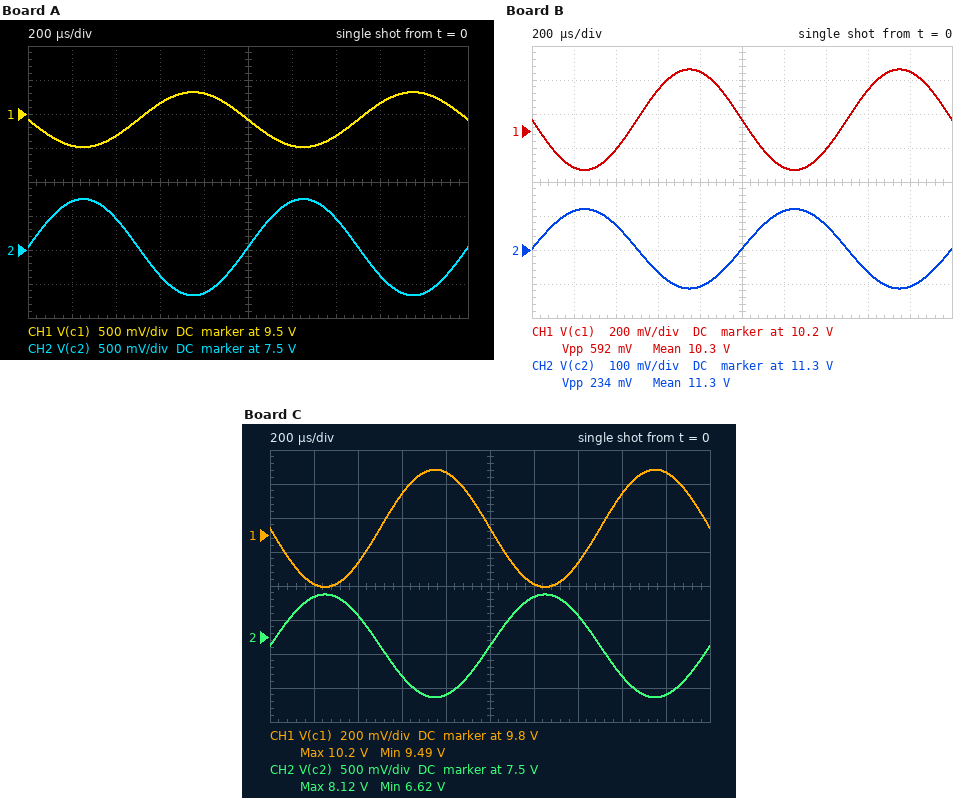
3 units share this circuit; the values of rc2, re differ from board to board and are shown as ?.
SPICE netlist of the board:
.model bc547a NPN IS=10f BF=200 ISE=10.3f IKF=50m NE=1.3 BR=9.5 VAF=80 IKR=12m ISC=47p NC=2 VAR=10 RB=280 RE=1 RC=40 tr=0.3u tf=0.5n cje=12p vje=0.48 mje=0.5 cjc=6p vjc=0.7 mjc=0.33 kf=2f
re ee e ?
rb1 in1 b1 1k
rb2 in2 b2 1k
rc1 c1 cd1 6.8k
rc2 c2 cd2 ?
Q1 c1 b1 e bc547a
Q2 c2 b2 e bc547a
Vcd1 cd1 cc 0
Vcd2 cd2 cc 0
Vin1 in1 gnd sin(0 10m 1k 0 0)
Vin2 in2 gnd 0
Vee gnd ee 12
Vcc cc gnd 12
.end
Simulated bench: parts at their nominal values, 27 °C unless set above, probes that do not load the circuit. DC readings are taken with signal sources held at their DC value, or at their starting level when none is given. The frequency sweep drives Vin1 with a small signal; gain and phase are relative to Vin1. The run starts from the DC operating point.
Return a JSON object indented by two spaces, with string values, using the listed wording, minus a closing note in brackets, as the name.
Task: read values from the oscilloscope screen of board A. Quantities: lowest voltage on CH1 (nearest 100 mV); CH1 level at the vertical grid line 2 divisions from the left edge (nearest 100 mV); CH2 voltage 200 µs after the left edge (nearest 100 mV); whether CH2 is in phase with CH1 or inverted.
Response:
{
  "lowest voltage on CH1": "9.0 V",
  "CH1 level at the vertical grid line 2 divisions from the left edge": "9.2 V",
  "CH2 voltage 200 µs after the left edge": "8.2 V",
  "whether CH2 is in phase with CH1 or inverted": "inverted"
}
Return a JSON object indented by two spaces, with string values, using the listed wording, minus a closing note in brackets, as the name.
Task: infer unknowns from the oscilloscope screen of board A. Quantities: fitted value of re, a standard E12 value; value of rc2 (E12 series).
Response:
{
  "fitted value of re, a standard E12 value": "15 kΩ",
  "value of rc2": "12 kΩ"
}
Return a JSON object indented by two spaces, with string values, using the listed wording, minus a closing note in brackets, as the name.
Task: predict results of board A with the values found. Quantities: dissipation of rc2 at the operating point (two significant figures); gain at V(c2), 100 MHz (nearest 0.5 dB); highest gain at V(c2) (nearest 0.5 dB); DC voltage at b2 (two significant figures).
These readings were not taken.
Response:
{
  "dissipation of rc2 at the operating point": "1.7 mW",
  "gain at V(c2), 100 MHz": "-10.0 dB",
  "highest gain at V(c2)": "37.0 dB",
  "DC voltage at b2": "-3.2 mV"
}
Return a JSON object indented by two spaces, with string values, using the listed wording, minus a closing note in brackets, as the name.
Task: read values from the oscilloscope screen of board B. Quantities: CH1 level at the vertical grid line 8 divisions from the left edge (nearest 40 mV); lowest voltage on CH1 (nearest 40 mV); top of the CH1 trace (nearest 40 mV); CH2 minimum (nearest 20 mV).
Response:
{
  "CH1 level at the vertical grid line 8 divisions from the left edge": "10.44 V",
  "lowest voltage on CH1": "9.96 V",
  "top of the CH1 trace": "10.56 V",
  "CH2 minimum": "11.18 V"
}
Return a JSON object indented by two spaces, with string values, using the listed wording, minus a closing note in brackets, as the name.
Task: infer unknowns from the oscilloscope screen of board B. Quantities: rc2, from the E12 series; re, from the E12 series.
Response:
{
  "rc2, from the E12 series": "2.7 kΩ",
  "re, from the E12 series": "22 kΩ"
}
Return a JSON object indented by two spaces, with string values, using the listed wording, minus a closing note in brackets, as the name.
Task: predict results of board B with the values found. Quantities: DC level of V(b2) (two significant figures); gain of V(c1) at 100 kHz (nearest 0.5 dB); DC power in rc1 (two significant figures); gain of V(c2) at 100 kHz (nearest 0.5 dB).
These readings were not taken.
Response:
{
  "DC level of V(b2)": "-2.2 mV",
  "gain of V(c1) at 100 kHz": "29.5 dB",
  "DC power in rc1": "440 µW",
  "gain of V(c2) at 100 kHz": "21.5 dB"
}
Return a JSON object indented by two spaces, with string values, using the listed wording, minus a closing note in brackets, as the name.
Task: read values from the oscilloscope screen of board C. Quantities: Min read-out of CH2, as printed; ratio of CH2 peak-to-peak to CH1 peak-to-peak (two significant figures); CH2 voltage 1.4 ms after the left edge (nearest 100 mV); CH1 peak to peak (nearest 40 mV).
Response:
{
  "Min read-out of CH2, as printed": "6.62 V",
  "ratio of CH2 peak-to-peak to CH1 peak-to-peak": "2.2",
  "CH2 voltage 1.4 ms after the left edge": "7.8 V",
  "CH1 peak to peak": "680 mV"
}
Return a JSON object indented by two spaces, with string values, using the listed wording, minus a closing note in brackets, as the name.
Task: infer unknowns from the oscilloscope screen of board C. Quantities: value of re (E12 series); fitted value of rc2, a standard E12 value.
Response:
{
  "value of re": "18 kΩ",
  "fitted value of rc2, a standard E12 value": "15 kΩ"
}
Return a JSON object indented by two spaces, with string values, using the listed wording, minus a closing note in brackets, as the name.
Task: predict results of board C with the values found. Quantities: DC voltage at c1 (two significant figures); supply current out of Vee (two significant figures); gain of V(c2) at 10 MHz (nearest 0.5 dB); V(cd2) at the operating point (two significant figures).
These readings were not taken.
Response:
{
  "DC voltage at c1": "9.8 V",
  "supply current out of Vee": "630 µA",
  "gain of V(c2) at 10 MHz": "5.5 dB",
  "V(cd2) at the operating point": "12 V"
}
